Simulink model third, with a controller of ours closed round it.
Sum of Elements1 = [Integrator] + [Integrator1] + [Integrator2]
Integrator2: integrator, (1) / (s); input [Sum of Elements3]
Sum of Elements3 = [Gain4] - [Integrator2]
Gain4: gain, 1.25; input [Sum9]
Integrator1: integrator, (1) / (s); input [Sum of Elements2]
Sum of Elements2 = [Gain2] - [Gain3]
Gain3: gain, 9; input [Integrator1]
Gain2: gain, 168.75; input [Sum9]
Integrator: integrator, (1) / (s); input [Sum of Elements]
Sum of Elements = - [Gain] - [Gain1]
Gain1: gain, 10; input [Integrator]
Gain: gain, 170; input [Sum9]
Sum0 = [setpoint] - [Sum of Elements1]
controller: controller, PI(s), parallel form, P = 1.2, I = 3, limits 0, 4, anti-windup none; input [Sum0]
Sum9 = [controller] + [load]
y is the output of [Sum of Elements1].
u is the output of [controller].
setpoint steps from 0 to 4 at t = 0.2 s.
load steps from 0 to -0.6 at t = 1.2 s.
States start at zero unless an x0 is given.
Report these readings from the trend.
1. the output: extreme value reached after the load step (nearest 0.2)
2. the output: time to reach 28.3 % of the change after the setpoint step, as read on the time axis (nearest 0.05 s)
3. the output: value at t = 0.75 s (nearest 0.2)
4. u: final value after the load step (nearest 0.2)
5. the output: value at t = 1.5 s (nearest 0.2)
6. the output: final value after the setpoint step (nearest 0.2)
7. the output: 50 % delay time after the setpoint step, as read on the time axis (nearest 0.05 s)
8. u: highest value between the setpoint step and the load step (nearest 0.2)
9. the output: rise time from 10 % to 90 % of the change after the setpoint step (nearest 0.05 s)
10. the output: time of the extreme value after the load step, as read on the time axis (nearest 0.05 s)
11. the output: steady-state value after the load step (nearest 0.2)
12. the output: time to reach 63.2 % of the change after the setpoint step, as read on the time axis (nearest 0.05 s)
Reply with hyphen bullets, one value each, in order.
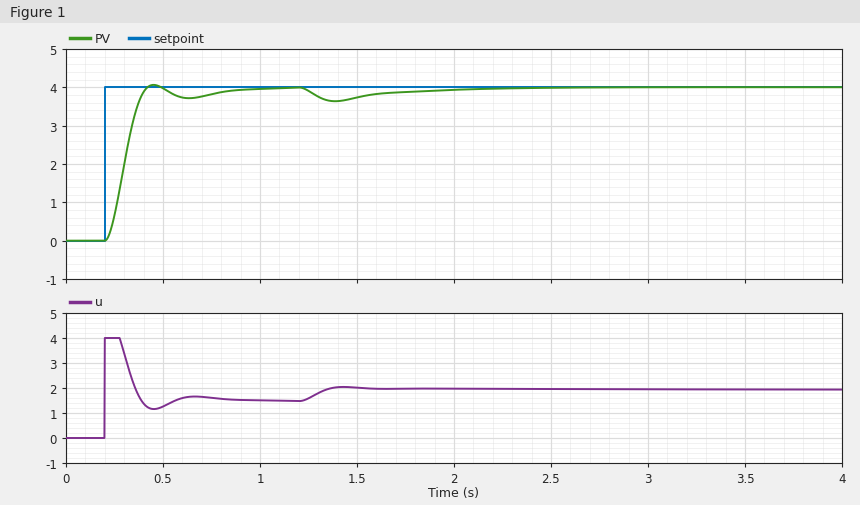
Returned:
- 3.6
- 0.25 s
- 3.8
- 2.0
- 3.8
- 4.0
- 0.30 s
- 4.0
- 0.15 s
- 1.40 s
- 4.0
- 0.30 s
